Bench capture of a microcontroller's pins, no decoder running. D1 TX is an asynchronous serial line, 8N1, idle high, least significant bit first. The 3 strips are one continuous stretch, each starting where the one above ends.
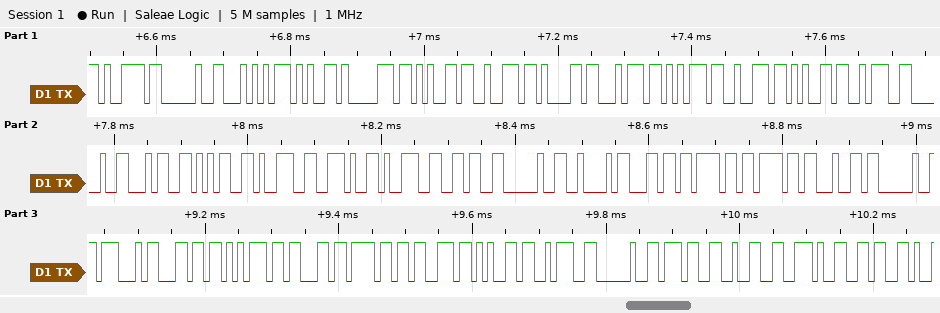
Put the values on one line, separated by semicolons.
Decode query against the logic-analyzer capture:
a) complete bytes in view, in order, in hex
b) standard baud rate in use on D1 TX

79 20 54 65 70 65 72 61 74 75 72 65 3A 20 34 35 39 2E 39 36 20 42 6C 6F 6F 64 20 47 6C 75 63 6F 73 65 3A 20 37 32 2E 36; 115200 baud
